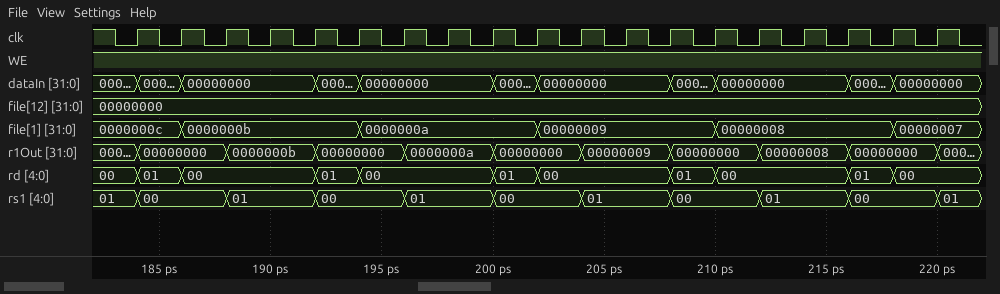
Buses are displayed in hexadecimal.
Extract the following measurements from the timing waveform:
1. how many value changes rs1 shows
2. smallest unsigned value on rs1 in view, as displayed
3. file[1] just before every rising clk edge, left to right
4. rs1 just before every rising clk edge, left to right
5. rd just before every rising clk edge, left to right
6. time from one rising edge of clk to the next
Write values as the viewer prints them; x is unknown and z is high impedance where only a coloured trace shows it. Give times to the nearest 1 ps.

10
00
0000000c, 0000000c, 0000000b, 0000000b, 0000000b, 0000000b, 0000000a, 0000000a, 0000000a, 0000000a, 00000009, 00000009, 00000009, 00000009, 00000008, 00000008, 00000008, 00000008, 00000007
01, 00, 00, 01, 01, 00, 00, 01, 01, 00, 00, 01, 01, 00, 00, 01, 01, 00, 00
00, 01, 00, 00, 00, 01, 00, 00, 00, 01, 00, 00, 00, 01, 00, 00, 00, 01, 00
2 ps
